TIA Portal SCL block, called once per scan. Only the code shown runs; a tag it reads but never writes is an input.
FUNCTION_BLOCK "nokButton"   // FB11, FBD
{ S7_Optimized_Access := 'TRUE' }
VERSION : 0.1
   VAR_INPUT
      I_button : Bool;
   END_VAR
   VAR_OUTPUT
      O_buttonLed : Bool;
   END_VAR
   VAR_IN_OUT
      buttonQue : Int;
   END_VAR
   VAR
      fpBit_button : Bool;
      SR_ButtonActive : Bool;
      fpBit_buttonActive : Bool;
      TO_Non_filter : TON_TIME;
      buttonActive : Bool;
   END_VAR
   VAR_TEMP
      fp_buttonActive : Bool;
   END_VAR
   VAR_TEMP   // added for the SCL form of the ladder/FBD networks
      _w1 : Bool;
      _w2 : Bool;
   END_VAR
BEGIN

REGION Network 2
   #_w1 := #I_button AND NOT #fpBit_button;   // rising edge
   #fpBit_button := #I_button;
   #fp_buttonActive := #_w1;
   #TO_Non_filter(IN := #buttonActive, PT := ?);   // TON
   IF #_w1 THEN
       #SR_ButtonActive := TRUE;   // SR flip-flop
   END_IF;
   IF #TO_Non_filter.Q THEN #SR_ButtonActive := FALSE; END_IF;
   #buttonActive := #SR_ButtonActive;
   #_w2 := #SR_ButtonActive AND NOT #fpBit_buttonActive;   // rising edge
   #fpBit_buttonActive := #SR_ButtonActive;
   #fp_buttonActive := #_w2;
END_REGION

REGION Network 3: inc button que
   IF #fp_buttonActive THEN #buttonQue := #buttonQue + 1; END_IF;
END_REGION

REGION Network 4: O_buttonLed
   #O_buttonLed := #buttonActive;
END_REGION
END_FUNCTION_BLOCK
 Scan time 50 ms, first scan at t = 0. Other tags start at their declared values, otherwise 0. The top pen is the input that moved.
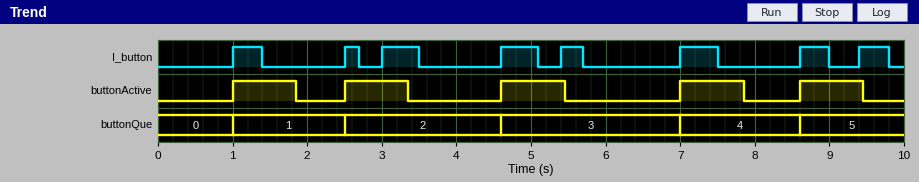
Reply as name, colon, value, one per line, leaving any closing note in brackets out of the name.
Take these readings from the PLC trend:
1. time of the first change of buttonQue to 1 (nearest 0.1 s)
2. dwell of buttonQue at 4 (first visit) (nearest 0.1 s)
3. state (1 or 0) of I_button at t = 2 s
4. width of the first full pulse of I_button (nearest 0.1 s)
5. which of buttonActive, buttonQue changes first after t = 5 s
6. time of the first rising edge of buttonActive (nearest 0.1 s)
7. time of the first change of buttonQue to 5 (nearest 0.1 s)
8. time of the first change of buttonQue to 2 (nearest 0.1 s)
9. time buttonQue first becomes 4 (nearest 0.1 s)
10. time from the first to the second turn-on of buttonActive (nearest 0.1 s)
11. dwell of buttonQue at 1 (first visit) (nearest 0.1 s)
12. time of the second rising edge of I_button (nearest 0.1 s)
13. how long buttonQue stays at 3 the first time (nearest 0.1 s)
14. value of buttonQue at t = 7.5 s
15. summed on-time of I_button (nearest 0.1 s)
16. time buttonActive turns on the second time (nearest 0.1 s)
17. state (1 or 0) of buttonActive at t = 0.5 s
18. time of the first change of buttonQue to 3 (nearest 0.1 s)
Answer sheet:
time of the first change of buttonQue to 1: 1.0 s
dwell of buttonQue at 4 (first visit): 1.6 s
state (1 or 0) of I_button at t = 2 s: 0
width of the first full pulse of I_button: 0.4 s
which of buttonActive, buttonQue changes first after t = 5 s: buttonActive
time of the first rising edge of buttonActive: 1.0 s
time of the first change of buttonQue to 5: 8.6 s
time of the first change of buttonQue to 2: 2.5 s
time buttonQue first becomes 4: 7.0 s
time from the first to the second turn-on of buttonActive: 1.5 s
dwell of buttonQue at 1 (first visit): 1.5 s
time of the second rising edge of I_button: 2.5 s
how long buttonQue stays at 3 the first time: 2.4 s
value of buttonQue at t = 7.5 s: 4
summed on-time of I_button: 3.2 s
time buttonActive turns on the second time: 2.5 s
state (1 or 0) of buttonActive at t = 0.5 s: 0
time of the first change of buttonQue to 3: 4.6 s
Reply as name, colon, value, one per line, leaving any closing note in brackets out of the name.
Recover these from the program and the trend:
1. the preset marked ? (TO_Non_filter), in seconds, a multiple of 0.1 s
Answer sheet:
the preset marked ? (TO_Non_filter), in seconds, a multiple of 0.1 s: 0.8 s
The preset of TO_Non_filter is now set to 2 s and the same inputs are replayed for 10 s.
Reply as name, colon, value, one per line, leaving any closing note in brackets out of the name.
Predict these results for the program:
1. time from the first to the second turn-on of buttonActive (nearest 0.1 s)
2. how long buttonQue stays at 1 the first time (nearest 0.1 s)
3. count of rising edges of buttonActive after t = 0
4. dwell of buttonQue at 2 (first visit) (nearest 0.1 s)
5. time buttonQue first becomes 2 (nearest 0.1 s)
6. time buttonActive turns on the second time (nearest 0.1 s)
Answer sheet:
time from the first to the second turn-on of buttonActive: 3.6 s
how long buttonQue stays at 1 the first time: 3.6 s
count of rising edges of buttonActive after t = 0: 4
dwell of buttonQue at 2 (first visit): 2.4 s
time buttonQue first becomes 2: 4.6 s
time buttonActive turns on the second time: 4.6 s
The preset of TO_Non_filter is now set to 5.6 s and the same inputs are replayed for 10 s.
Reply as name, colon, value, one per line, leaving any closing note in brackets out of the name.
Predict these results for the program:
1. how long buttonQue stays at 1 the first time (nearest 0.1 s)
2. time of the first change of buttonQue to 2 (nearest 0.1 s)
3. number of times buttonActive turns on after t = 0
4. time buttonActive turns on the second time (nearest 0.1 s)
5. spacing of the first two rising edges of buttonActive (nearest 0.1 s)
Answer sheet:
how long buttonQue stays at 1 the first time: 6.0 s
time of the first change of buttonQue to 2: 7.0 s
number of times buttonActive turns on after t = 0: 2
time buttonActive turns on the second time: 7.0 s
spacing of the first two rising edges of buttonActive: 6.0 s
